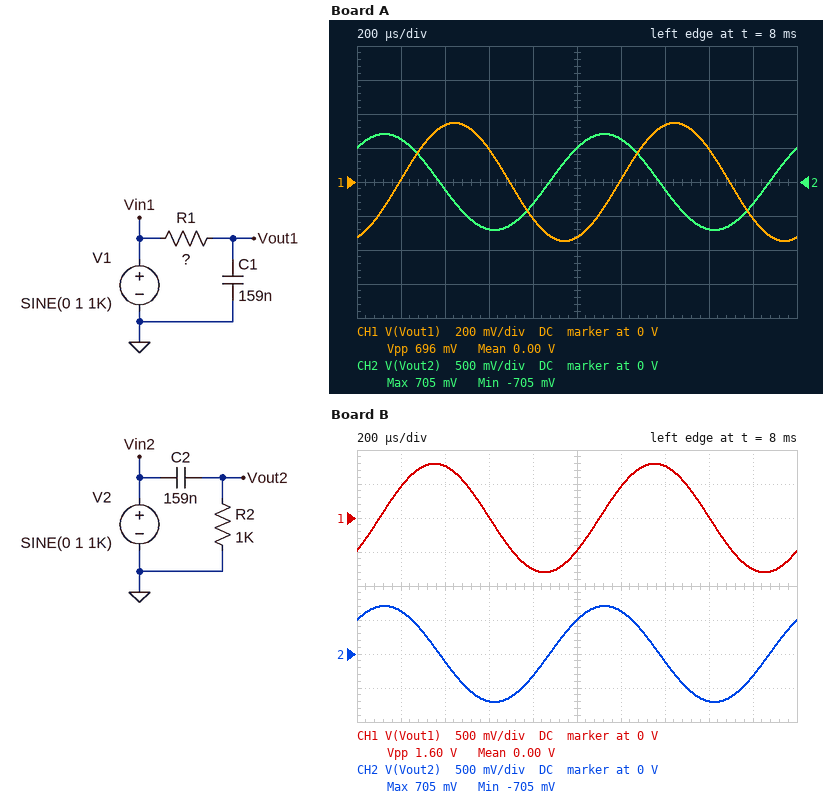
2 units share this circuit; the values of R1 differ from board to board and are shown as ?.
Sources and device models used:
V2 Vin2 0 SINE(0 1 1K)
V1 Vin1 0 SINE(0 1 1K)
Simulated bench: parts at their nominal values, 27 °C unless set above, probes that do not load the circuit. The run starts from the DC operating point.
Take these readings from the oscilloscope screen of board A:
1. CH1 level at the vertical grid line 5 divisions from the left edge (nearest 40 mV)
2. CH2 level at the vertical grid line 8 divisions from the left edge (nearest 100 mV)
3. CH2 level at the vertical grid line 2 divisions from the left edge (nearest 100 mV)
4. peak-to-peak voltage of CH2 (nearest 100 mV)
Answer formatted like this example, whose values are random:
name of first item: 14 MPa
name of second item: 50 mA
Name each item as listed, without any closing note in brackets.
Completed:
CH1 level at the vertical grid line 5 divisions from the left edge: -320 mV
CH2 level at the vertical grid line 8 divisions from the left edge: -700 mV
CH2 level at the vertical grid line 2 divisions from the left edge: -100 mV
peak-to-peak voltage of CH2: 1.4 V
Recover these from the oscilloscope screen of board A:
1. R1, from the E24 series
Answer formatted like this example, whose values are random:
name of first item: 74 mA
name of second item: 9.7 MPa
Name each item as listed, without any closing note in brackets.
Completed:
R1, from the E24 series: 2.7 kΩ
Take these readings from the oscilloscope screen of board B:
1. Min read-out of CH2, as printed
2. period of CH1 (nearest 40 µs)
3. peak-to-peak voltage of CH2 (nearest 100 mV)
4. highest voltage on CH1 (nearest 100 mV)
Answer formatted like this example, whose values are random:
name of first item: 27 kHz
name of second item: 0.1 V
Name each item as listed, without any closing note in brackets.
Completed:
Min read-out of CH2, as printed: -705 mV
period of CH1: 1.00 ms
peak-to-peak voltage of CH2: 1.4 V
highest voltage on CH1: 800 mV
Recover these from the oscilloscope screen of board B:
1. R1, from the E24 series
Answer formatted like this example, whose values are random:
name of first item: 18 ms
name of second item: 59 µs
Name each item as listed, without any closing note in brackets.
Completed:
R1, from the E24 series: 750 Ω
